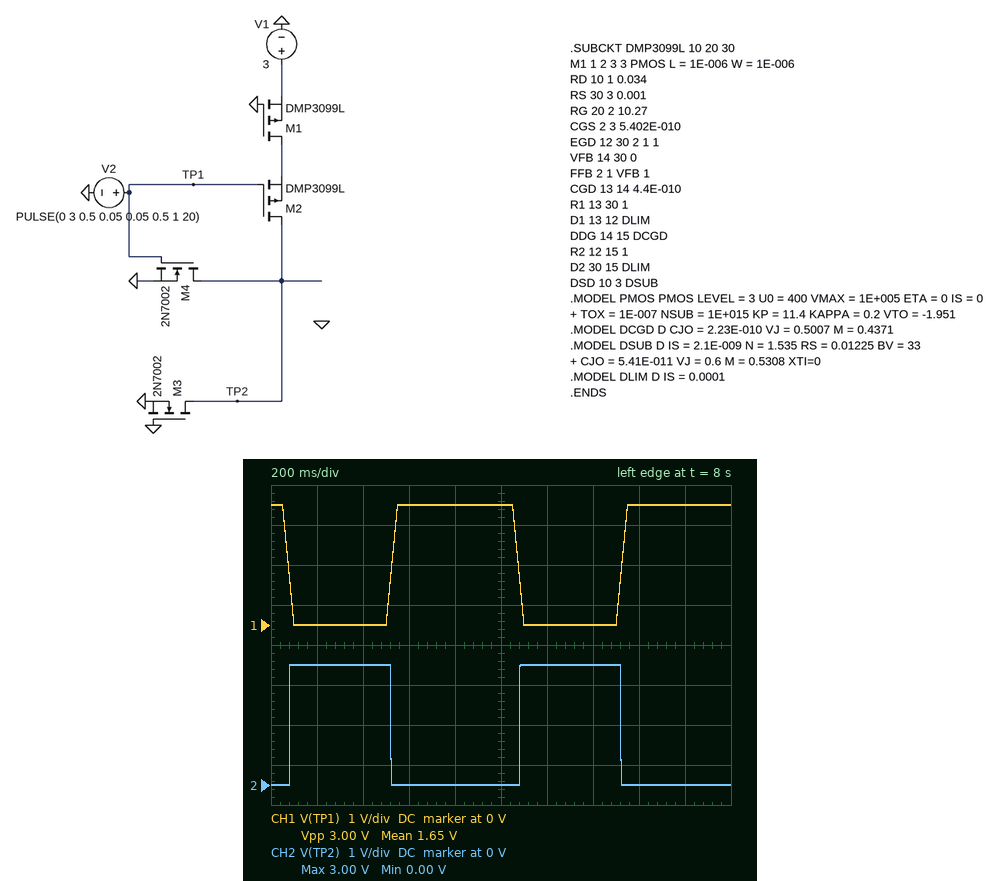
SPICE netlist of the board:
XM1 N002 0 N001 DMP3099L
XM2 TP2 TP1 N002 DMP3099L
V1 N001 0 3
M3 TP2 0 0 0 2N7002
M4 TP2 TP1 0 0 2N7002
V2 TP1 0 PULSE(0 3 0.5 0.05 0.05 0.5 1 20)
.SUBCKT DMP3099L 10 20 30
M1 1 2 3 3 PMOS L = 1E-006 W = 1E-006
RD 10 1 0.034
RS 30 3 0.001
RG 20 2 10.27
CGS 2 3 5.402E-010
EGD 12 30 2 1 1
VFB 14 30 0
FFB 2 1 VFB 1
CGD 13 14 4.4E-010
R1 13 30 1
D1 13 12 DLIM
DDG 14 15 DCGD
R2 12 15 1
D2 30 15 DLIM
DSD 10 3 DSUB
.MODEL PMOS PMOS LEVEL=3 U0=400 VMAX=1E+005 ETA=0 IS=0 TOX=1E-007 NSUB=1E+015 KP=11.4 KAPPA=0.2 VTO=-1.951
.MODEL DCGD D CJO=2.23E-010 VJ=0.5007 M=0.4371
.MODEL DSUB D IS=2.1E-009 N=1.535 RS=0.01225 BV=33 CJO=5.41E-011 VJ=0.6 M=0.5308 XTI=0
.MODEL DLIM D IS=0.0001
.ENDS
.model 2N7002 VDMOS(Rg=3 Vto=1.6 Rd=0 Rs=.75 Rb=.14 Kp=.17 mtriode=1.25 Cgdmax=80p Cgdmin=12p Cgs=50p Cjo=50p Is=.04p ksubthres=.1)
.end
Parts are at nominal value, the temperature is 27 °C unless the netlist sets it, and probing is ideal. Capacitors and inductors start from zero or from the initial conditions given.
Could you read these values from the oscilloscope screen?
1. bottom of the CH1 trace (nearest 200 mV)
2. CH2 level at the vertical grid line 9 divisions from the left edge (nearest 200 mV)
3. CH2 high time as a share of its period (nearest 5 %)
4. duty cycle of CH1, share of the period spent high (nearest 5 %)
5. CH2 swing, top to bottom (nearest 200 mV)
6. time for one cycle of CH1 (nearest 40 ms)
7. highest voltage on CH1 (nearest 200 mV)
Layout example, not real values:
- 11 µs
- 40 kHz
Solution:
- 0 V
- 0 V
- 45 %
- 55 %
- 3.0 V
- 1.00 s
- 3.0 V
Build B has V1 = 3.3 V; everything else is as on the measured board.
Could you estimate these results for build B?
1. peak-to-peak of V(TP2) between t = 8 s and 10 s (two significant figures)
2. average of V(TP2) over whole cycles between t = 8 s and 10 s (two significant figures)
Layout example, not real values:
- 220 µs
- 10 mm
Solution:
- 3.3 V
- 1.5 V
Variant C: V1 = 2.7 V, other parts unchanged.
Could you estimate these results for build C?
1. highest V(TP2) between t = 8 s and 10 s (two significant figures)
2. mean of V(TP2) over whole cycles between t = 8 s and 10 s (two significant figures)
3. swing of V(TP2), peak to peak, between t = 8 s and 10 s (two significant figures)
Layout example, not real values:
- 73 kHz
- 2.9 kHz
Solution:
- 2.8 V
- 1.2 V
- 2.9 V
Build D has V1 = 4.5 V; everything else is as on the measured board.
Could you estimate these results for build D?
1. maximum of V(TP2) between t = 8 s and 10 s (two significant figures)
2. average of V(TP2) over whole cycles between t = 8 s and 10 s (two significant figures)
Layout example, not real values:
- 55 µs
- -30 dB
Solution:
- 4.5 V
- 2.2 V
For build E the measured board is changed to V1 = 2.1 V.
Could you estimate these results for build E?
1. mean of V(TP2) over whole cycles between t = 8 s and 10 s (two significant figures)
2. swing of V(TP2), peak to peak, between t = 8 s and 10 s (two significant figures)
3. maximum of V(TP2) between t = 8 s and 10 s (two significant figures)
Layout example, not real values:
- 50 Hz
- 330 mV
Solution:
- 890 mV
- 2.5 V
- 2.2 V
